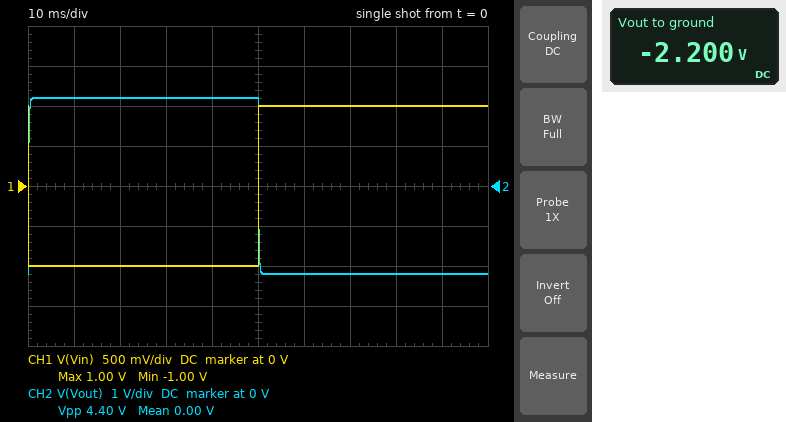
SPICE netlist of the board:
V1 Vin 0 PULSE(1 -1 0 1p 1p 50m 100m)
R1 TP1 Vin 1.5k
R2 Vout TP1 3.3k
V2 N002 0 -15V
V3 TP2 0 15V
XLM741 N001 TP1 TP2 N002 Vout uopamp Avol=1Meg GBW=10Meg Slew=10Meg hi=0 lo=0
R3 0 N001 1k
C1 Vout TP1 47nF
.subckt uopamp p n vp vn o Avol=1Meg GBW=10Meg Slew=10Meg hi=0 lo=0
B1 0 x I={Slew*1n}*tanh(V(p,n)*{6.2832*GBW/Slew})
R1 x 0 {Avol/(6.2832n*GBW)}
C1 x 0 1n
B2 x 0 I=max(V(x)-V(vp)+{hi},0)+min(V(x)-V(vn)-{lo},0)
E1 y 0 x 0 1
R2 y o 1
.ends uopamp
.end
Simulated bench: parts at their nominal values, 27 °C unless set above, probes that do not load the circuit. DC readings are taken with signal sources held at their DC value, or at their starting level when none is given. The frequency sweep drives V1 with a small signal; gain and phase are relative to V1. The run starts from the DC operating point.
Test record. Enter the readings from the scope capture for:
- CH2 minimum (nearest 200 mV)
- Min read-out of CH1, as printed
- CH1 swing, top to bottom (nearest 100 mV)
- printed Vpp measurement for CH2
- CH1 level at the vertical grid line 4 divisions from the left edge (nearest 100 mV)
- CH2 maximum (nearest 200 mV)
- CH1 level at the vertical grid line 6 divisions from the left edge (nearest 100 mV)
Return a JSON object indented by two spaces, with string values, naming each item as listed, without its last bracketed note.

{
  "CH2 minimum": "-2.2 V",
  "Min read-out of CH1, as printed": "-1.00 V",
  "CH1 swing, top to bottom": "2.0 V",
  "printed Vpp measurement for CH2": "4.40 V",
  "CH1 level at the vertical grid line 4 divisions from the left edge": "-1.0 V",
  "CH2 maximum": "2.2 V",
  "CH1 level at the vertical grid line 6 divisions from the left edge": "1.0 V"
}
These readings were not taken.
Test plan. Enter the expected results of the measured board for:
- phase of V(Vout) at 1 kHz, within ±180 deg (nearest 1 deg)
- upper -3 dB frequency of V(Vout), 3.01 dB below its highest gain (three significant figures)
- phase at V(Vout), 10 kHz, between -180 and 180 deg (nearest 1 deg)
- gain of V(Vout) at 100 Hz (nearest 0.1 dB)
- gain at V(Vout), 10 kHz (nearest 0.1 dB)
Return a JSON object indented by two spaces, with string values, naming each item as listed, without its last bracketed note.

{
  "phase of V(Vout) at 1 kHz, within ±180 deg": "136 deg",
  "upper -3 dB frequency of V(Vout), 3.01 dB below its highest gain": "1.03 kHz",
  "phase at V(Vout), 10 kHz, between -180 and 180 deg": "96 deg",
  "gain of V(Vout) at 100 Hz": "6.8 dB",
  "gain at V(Vout), 10 kHz": "-13.0 dB"
}
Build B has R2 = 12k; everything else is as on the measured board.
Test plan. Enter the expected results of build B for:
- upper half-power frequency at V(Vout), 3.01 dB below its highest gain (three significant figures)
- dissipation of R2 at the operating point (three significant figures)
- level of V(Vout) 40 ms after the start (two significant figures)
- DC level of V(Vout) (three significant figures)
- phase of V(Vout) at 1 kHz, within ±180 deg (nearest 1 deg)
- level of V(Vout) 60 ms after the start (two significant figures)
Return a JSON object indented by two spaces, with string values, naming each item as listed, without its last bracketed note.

{
  "upper half-power frequency at V(Vout), 3.01 dB below its highest gain": "282 Hz",
  "dissipation of R2 at the operating point": "5.33 mW",
  "level of V(Vout) 40 ms after the start": "8.0 V",
  "DC level of V(Vout)": "-8.00 V",
  "phase of V(Vout) at 1 kHz, within ±180 deg": "106 deg",
  "level of V(Vout) 60 ms after the start": "-8.0 V"
}
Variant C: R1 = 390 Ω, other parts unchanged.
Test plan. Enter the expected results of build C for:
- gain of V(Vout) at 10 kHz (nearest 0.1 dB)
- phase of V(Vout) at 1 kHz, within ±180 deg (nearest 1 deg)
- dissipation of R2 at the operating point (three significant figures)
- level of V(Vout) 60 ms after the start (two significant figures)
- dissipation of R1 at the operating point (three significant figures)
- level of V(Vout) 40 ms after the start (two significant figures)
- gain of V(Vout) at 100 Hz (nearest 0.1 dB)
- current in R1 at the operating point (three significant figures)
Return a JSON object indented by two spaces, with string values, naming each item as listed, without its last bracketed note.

{
  "gain of V(Vout) at 10 kHz": "-1.3 dB",
  "phase of V(Vout) at 1 kHz, within ±180 deg": "136 deg",
  "dissipation of R2 at the operating point": "21.7 mW",
  "level of V(Vout) 60 ms after the start": "-8.5 V",
  "dissipation of R1 at the operating point": "2.56 mW",
  "level of V(Vout) 40 ms after the start": "8.5 V",
  "gain of V(Vout) at 100 Hz": "18.5 dB",
  "current in R1 at the operating point": "2.56 mA"
}
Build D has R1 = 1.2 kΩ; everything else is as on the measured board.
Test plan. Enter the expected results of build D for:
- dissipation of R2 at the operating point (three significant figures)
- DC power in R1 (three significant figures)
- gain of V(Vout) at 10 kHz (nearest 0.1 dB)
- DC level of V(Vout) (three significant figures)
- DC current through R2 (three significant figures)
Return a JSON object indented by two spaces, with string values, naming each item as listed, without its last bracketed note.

{
  "dissipation of R2 at the operating point": "2.29 mW",
  "DC power in R1": "833 µW",
  "gain of V(Vout) at 10 kHz": "-11.0 dB",
  "DC level of V(Vout)": "-2.75 V",
  "DC current through R2": "833 µA"
}
